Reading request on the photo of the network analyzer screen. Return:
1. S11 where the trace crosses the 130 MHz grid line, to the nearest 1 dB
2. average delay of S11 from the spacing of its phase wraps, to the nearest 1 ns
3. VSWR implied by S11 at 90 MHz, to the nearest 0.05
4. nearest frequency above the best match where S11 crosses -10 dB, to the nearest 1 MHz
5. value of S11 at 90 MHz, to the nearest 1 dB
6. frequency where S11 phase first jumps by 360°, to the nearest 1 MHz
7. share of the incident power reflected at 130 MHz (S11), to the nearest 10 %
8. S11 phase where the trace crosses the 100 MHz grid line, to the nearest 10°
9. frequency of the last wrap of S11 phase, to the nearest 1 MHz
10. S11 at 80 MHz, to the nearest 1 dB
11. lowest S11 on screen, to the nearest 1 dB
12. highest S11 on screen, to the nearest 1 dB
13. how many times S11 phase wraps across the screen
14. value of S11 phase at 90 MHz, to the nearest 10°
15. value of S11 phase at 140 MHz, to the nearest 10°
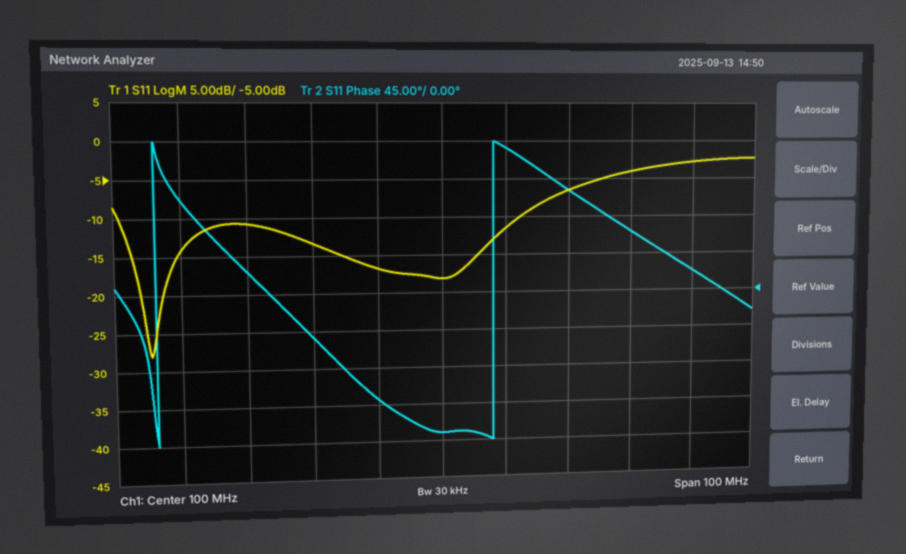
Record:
-4 dB
19 ns
1.35
112 MHz
-17 dB
56 MHz
40 %
-170°
108 MHz
-13 dB
-28 dB
-2 dB
2
-130°
20°
